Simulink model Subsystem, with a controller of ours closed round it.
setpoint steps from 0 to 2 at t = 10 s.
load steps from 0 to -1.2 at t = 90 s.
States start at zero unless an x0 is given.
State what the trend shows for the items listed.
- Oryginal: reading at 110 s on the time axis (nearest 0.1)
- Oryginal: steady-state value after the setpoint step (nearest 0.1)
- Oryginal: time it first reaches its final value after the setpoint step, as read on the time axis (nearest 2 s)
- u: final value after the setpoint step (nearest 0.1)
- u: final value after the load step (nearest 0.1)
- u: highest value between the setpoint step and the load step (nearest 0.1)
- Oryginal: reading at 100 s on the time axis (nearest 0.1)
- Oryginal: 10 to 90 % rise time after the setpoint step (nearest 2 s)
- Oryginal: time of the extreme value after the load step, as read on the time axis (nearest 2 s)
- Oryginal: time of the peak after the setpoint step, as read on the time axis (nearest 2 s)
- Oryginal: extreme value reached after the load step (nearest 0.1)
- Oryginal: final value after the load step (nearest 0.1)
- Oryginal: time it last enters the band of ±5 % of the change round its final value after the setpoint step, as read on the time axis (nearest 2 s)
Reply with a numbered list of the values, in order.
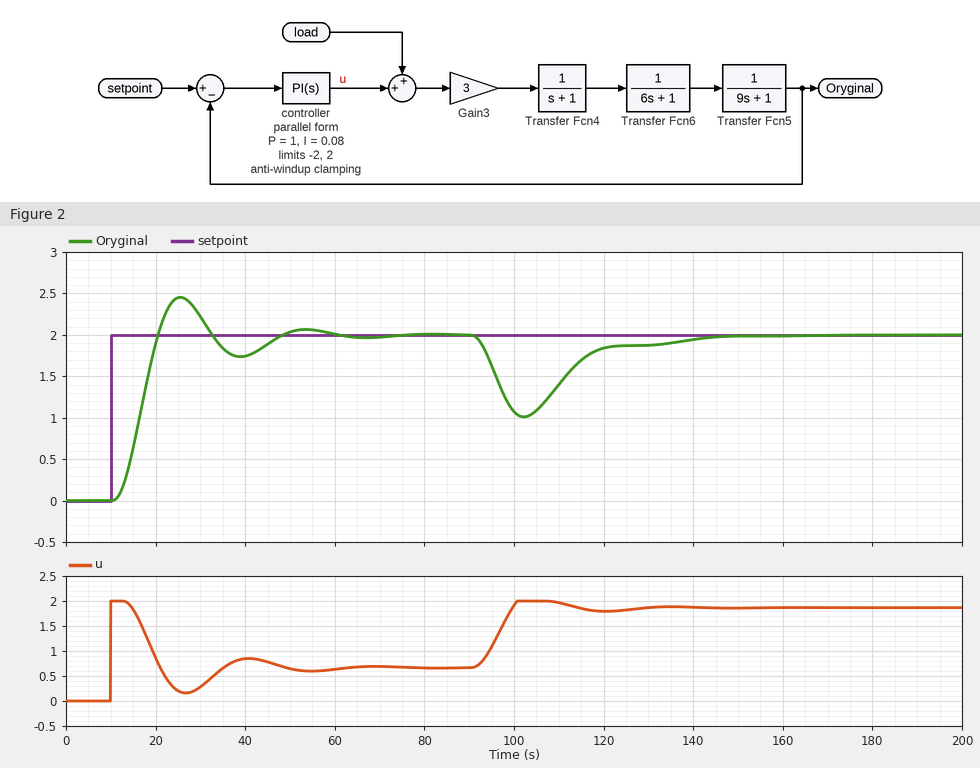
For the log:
1. 1.4
2. 2.0
3. 20 s
4. 0.7
5. 1.9
6. 2.0
7. 1.1
8. 6 s
9. 102 s
10. 26 s
11. 1.0
12. 2.0
13. 46 s
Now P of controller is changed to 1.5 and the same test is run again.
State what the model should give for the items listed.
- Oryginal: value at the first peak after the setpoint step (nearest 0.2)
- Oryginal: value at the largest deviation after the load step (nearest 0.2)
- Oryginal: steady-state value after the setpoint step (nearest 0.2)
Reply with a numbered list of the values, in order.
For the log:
1. 2.2
2. 1.2
3. 2.0
